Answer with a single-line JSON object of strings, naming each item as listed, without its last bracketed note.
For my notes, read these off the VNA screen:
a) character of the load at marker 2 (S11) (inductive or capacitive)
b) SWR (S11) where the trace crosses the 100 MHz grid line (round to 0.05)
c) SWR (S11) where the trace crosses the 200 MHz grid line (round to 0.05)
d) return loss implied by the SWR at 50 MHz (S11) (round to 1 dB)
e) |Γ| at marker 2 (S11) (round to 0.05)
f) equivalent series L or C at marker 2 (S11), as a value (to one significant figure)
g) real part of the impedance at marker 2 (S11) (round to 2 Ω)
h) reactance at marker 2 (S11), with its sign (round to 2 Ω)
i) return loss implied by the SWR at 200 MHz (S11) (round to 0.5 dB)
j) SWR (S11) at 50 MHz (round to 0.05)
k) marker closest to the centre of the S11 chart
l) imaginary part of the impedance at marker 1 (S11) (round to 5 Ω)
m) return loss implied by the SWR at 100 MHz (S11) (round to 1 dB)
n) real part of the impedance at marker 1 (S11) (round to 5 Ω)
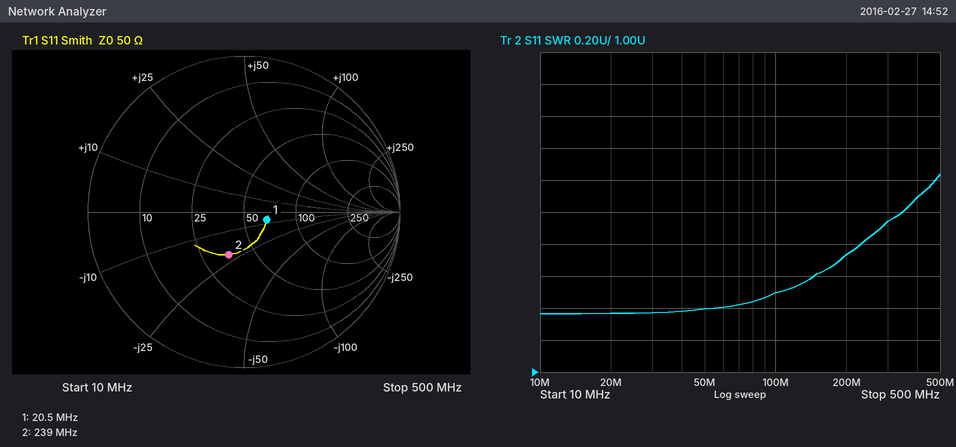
{"character of the load at marker 2 (S11)": "capacitive", "SWR (S11) where the trace crosses the 100 MHz grid line": "1.50", "SWR (S11) where the trace crosses the 200 MHz grid line": "1.75", "return loss implied by the SWR at 50 MHz (S11)": "16 dB", "|Γ| at marker 2 (S11)": "0.30", "equivalent series L or C at marker 2 (S11), as a value": "30 pF", "real part of the impedance at marker 2 (S11)": "36 Ω", "reactance at marker 2 (S11), with its sign": "-22 Ω", "return loss implied by the SWR at 200 MHz (S11)": "11.5 dB", "SWR (S11) at 50 MHz": "1.40", "marker closest to the centre of the S11 chart": "marker 1", "imaginary part of the impedance at marker 1 (S11)": "-5 Ω", "return loss implied by the SWR at 100 MHz (S11)": "14 dB", "real part of the impedance at marker 1 (S11)": "65 Ω"}
